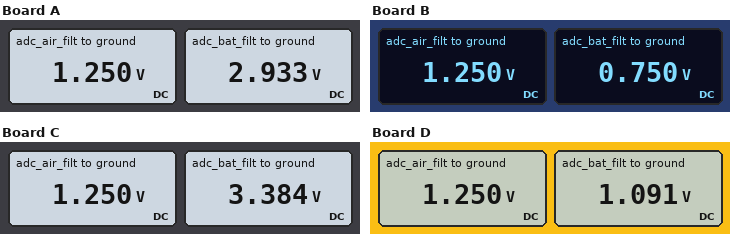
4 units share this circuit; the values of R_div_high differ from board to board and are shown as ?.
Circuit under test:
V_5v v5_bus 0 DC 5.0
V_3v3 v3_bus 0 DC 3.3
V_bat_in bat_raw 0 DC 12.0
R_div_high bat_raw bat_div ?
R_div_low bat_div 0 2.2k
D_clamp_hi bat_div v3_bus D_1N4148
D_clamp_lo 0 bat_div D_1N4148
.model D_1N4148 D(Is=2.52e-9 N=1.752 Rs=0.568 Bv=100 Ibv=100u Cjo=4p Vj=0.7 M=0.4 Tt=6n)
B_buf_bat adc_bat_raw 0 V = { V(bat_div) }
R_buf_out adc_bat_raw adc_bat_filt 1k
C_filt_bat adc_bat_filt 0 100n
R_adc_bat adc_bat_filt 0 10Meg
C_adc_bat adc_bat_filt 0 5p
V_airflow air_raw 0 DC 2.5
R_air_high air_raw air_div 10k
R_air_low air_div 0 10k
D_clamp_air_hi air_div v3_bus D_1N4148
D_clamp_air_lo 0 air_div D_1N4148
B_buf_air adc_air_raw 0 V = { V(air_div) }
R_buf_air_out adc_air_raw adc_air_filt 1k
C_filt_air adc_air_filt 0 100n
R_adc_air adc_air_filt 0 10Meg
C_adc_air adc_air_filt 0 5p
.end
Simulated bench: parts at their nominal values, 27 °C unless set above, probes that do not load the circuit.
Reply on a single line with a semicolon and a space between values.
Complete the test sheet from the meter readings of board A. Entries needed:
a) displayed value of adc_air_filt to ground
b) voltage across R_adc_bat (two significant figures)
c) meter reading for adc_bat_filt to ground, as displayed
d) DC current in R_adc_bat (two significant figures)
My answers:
1.250 V; 2.9 V; 2.933 V; 290 nA
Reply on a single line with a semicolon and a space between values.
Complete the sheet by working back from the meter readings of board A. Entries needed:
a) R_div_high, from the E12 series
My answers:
6.8 kΩ
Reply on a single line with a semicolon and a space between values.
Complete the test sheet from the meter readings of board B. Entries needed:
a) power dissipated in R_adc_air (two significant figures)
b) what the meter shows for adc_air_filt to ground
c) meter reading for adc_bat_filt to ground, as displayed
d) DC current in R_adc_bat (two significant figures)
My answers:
160 nW; 1.250 V; 0.750 V; 75 nA
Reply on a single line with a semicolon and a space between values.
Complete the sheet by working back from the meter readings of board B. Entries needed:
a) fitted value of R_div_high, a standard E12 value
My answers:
33 kΩ
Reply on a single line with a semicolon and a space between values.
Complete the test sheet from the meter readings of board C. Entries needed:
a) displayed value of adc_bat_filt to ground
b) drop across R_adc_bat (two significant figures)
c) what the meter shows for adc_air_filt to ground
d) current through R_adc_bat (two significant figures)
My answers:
3.384 V; 3.4 V; 1.250 V; 340 nA
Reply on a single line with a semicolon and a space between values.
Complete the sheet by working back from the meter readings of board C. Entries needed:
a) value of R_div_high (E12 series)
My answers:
5.6 kΩ
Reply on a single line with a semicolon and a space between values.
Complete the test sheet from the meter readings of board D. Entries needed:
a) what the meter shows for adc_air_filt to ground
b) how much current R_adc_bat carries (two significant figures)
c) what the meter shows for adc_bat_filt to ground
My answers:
1.250 V; 110 nA; 1.091 V
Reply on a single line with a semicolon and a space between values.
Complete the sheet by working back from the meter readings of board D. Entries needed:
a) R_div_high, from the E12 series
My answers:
22 kΩ
